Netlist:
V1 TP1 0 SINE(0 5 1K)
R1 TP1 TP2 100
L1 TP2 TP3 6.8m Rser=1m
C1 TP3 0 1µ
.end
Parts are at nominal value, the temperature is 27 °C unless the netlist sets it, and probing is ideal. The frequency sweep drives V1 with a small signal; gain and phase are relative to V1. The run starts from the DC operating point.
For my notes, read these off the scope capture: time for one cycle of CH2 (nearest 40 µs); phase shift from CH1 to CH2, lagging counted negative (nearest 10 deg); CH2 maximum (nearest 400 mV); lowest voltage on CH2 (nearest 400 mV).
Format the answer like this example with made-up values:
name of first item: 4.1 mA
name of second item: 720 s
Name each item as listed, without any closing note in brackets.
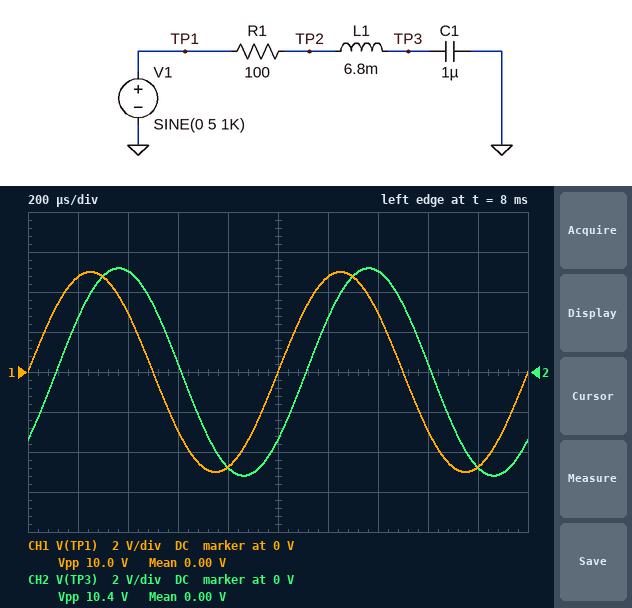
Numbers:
time for one cycle of CH2: 1.00 ms
phase shift from CH1 to CH2, lagging counted negative: -40 deg
CH2 maximum: 5.2 V
lowest voltage on CH2: -5.2 V
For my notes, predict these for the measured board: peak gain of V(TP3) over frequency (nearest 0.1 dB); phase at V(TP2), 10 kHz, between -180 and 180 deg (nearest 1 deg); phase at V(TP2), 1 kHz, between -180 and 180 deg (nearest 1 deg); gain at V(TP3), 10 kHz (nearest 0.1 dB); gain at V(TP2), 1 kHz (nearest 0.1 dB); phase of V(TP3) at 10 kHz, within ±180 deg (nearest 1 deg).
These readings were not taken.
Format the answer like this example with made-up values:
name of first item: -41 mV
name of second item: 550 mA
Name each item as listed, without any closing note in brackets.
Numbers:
peak gain of V(TP3) over frequency: 0.3 dB
phase at V(TP2), 10 kHz, between -180 and 180 deg: 14 deg
phase at V(TP2), 1 kHz, between -180 and 180 deg: -41 deg
gain at V(TP3), 10 kHz: -28.5 dB
gain at V(TP2), 1 kHz: -2.4 dB
phase of V(TP3) at 10 kHz, within ±180 deg: -166 deg
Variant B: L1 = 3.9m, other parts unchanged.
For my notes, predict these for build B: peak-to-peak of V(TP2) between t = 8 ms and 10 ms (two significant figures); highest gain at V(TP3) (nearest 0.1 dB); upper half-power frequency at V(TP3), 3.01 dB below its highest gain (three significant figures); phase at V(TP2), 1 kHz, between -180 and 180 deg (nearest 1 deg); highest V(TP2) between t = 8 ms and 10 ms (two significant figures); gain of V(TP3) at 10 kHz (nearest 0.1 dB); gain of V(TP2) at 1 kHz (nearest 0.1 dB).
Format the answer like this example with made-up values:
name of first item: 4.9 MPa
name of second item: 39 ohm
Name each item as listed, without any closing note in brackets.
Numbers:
peak-to-peak of V(TP2) between t = 8 ms and 10 ms: 8.0 V
highest gain at V(TP3): 0 dB
upper half-power frequency at V(TP3), 3.01 dB below its highest gain: 2.22 kHz
phase at V(TP2), 1 kHz, between -180 and 180 deg: -37 deg
highest V(TP2) between t = 8 ms and 10 ms: 4.0 V
gain of V(TP3) at 10 kHz: -23.9 dB
gain of V(TP2) at 1 kHz: -1.9 dB
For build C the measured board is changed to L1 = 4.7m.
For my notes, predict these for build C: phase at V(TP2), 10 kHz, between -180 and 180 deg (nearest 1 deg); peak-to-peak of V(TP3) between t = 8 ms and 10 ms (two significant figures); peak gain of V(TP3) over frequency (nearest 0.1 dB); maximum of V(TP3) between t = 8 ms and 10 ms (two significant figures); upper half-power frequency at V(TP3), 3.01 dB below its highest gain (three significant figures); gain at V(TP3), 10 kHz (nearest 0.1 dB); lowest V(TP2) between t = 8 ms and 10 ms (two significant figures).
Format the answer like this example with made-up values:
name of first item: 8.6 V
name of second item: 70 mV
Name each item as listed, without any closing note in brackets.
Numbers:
phase at V(TP2), 10 kHz, between -180 and 180 deg: 20 deg
peak-to-peak of V(TP3) between t = 8 ms and 10 ms: 9.7 V
peak gain of V(TP3) over frequency: 0 dB
maximum of V(TP3) between t = 8 ms and 10 ms: 4.9 V
upper half-power frequency at V(TP3), 3.01 dB below its highest gain: 2.25 kHz
gain at V(TP3), 10 kHz: -25.4 dB
lowest V(TP2) between t = 8 ms and 10 ms: -4.0 V
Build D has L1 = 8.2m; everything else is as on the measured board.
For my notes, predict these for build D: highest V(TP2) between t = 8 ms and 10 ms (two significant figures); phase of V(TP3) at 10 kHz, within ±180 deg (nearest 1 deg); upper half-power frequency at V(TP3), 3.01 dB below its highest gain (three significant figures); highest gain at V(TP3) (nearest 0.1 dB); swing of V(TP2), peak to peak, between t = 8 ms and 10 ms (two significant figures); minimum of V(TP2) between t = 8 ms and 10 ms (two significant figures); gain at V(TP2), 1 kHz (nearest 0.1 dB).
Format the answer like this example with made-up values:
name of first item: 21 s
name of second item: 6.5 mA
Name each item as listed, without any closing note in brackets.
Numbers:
highest V(TP2) between t = 8 ms and 10 ms: 3.7 V
phase of V(TP3) at 10 kHz, within ±180 deg: -169 deg
upper half-power frequency at V(TP3), 3.01 dB below its highest gain: 2.01 kHz
highest gain at V(TP3): 0.7 dB
swing of V(TP2), peak to peak, between t = 8 ms and 10 ms: 7.3 V
minimum of V(TP2) between t = 8 ms and 10 ms: -3.7 V
gain at V(TP2), 1 kHz: -2.7 dB
